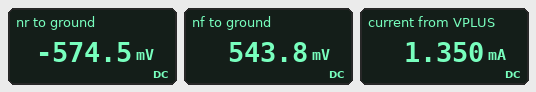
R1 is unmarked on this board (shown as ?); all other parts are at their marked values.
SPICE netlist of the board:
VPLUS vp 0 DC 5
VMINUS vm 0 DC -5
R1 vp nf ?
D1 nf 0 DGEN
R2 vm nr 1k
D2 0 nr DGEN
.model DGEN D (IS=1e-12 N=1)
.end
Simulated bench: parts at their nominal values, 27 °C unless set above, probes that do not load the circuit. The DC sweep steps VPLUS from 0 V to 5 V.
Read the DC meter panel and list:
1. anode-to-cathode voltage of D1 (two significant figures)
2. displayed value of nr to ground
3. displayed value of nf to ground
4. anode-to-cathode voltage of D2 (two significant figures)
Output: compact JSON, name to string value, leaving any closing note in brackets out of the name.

{"anode-to-cathode voltage of D1": "540 mV", "displayed value of nr to ground": "-574.5 mV", "displayed value of nf to ground": "543.8 mV", "anode-to-cathode voltage of D2": "570 mV"}
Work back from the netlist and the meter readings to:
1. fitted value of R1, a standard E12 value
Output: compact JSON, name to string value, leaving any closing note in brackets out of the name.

{"fitted value of R1, a standard E12 value": "3.3 kΩ"}
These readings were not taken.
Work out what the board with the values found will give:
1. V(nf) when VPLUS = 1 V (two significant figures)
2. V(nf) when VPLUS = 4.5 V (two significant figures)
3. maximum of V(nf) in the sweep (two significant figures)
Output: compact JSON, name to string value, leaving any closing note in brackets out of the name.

{"V(nf) when VPLUS = 1 V": "490 mV", "V(nf) when VPLUS = 4.5 V": "540 mV", "maximum of V(nf) in the sweep": "540 mV"}
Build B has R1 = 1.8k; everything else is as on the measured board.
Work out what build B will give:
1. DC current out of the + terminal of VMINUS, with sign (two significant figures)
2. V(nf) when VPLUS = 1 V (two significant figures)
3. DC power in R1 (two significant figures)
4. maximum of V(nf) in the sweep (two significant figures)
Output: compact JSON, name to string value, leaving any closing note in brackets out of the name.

{"DC current out of the + terminal of VMINUS, with sign": "-4.4 mA", "V(nf) when VPLUS = 1 V": "500 mV", "DC power in R1": "11 mW", "maximum of V(nf) in the sweep": "560 mV"}
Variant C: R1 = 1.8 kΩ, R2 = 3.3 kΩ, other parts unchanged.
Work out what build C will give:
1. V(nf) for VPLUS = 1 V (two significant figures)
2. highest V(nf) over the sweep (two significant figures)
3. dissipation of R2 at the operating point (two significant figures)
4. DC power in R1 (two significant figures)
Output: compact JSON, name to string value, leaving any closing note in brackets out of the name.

{"V(nf) for VPLUS = 1 V": "500 mV", "highest V(nf) over the sweep": "560 mV", "dissipation of R2 at the operating point": "6.0 mW", "DC power in R1": "11 mW"}
